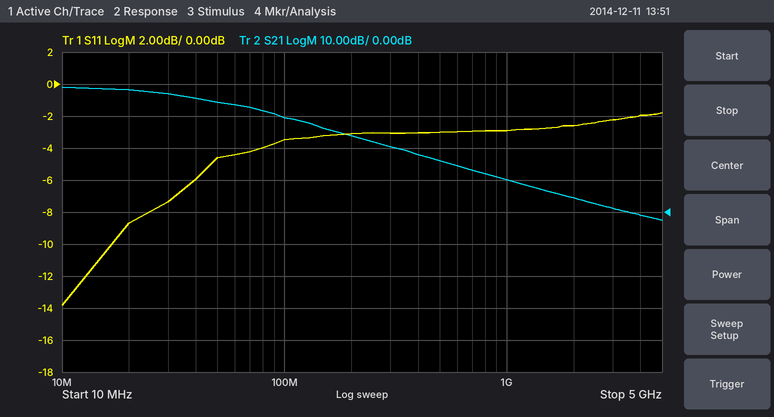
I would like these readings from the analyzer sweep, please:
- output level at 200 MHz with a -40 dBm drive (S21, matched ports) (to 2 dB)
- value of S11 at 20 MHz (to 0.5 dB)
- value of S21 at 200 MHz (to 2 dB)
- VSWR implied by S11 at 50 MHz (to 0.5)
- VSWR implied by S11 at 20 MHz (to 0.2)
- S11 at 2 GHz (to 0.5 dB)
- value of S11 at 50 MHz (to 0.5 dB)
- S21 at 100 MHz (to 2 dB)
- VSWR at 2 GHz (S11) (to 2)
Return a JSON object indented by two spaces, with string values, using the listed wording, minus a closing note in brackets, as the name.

{
  "output level at 200 MHz with a -40 dBm drive (S21, matched ports)": "-16 dBm",
  "value of S11 at 20 MHz": "-8.5 dB",
  "value of S21 at 200 MHz": "24 dB",
  "VSWR implied by S11 at 50 MHz": "4.0",
  "VSWR implied by S11 at 20 MHz": "2.2",
  "S11 at 2 GHz": "-2.5 dB",
  "value of S11 at 50 MHz": "-4.5 dB",
  "S21 at 100 MHz": "30 dB",
  "VSWR at 2 GHz (S11)": "6"
}
